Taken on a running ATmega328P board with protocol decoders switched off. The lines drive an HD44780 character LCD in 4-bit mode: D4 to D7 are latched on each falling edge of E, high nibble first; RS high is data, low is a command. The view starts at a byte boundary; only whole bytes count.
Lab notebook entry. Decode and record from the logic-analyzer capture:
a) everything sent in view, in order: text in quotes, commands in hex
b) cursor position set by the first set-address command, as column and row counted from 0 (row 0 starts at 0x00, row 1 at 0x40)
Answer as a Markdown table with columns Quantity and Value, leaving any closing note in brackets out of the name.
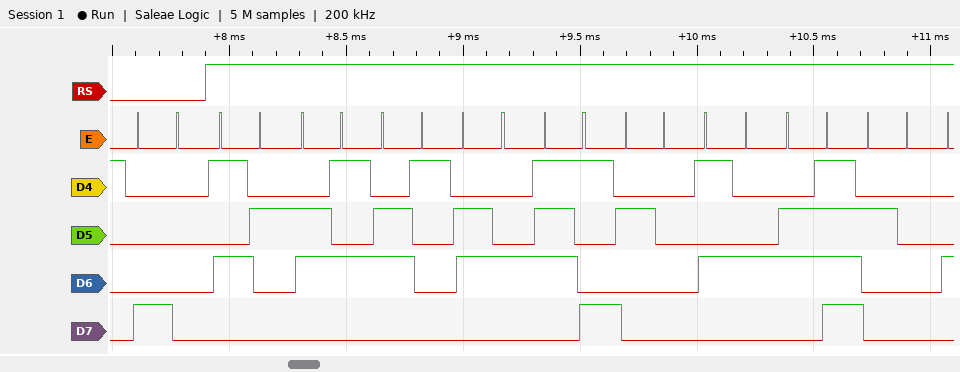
| Quantity | Value |
|---|---|
| everything sent in view, in order: text in quotes, commands in hex | 0x80 "Ready To " |
| cursor position set by the first set-address command, as column and row counted from 0 | column 0, row 0 |
